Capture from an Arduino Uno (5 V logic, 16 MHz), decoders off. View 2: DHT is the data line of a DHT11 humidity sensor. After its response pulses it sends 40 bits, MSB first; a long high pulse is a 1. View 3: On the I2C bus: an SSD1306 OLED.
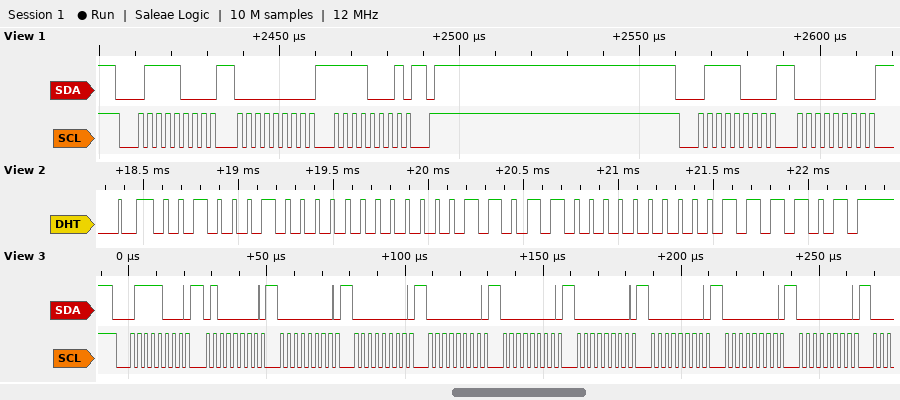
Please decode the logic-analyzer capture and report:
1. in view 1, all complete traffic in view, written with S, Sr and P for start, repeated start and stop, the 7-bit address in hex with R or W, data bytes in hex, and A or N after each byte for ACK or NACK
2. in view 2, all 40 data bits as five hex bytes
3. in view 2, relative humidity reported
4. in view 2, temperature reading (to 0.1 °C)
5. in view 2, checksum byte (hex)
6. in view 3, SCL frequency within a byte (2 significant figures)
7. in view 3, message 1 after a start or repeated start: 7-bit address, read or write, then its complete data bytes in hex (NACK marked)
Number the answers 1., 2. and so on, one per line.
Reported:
1. S 3CW A 00 A F1 A P S 3CW A 00 A
2. 22 00 1B 00 3D
3. 34 %
4. 27.0 °C
5. 0x3D
6. 400 kHz
7. 0x3C write: 40 00 00 00 00 00 00 00 00
